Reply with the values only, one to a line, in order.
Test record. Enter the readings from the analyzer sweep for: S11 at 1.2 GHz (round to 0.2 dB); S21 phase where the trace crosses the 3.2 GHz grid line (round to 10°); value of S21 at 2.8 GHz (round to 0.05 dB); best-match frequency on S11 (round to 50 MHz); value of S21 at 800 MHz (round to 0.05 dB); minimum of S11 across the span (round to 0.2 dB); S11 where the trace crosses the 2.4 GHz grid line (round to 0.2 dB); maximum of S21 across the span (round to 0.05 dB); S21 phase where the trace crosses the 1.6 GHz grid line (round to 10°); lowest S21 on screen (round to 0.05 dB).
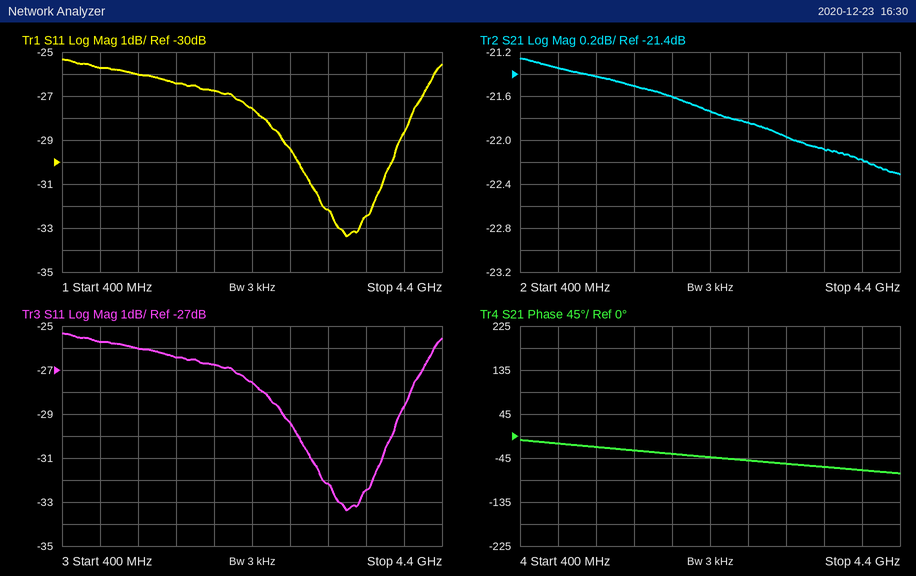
-26.0 dB
-60°
-21.85 dB
3.40 GHz
-21.35 dB
-33.4 dB
-27.6 dB
-21.25 dB
-30°
-22.30 dB
